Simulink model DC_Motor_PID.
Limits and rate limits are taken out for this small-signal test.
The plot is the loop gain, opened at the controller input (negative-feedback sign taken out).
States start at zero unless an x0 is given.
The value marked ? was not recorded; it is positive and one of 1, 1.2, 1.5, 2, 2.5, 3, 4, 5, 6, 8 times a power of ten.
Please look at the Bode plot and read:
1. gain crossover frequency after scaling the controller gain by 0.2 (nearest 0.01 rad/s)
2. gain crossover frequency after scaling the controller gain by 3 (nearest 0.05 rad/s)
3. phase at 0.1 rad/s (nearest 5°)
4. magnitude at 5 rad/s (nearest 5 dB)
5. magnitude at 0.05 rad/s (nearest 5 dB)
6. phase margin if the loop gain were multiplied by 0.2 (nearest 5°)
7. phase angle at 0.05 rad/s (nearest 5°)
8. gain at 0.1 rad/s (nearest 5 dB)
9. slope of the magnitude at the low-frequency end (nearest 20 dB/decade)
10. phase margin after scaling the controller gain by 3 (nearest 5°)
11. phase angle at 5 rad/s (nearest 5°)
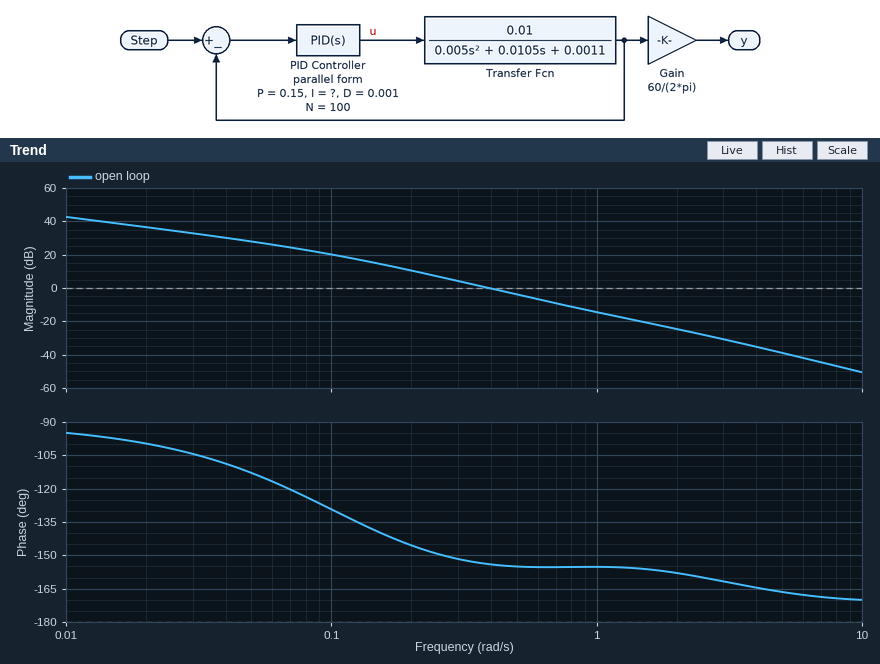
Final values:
0.16 rad/s
0.70 rad/s
-130°
-40 dB
30 dB
40°
-115°
20 dB
-20 dB/decade
25°
-165°
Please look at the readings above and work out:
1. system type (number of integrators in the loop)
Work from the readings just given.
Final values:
1
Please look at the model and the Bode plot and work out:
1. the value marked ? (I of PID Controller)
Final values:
0.15
